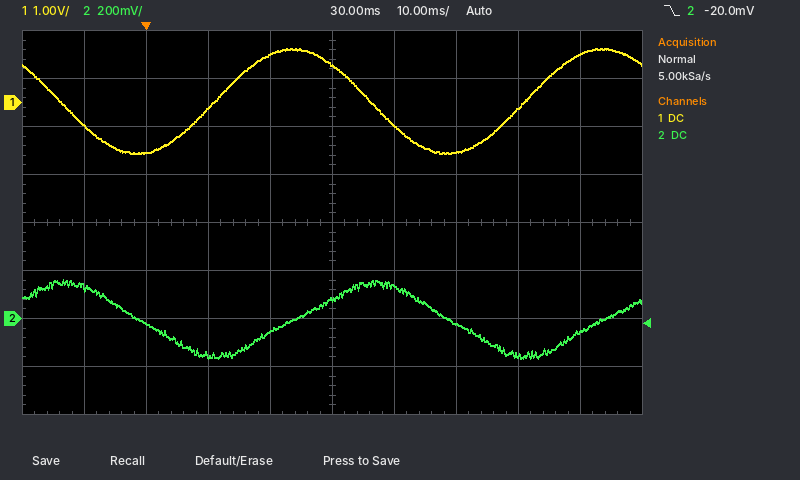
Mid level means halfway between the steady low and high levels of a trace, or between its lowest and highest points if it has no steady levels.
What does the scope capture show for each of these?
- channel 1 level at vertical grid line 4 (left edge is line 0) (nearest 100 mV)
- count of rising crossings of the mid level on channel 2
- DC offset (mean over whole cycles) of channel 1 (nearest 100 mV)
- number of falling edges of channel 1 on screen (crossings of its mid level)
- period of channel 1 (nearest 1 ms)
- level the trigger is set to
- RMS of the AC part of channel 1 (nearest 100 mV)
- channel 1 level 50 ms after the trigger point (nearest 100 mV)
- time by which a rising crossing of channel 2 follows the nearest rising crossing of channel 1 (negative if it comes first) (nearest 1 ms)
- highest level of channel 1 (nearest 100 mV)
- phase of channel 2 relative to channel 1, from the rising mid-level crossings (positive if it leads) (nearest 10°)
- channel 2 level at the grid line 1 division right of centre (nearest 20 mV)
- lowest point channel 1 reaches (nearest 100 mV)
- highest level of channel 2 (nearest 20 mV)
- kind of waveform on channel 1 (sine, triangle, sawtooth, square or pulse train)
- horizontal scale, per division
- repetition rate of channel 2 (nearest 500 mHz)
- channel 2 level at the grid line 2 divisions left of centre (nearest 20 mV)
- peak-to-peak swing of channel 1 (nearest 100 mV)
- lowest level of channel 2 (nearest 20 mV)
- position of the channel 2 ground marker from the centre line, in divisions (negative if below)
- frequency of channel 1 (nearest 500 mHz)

1.0 V
2
0.0 V
2
50 ms
-20.0 mV
800 mV
-1.0 V
+13 ms
1.1 V
-90°
140 mV
-1.1 V
160 mV
sine
10 ms
20.0 Hz
-160 mV
2.2 V
-160 mV
-2.0 div
20.0 Hz
